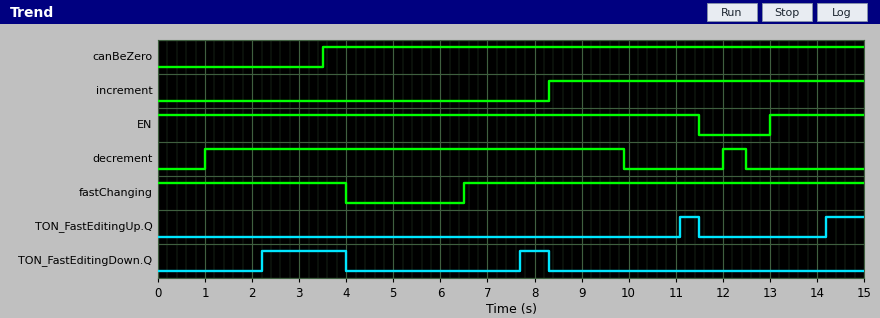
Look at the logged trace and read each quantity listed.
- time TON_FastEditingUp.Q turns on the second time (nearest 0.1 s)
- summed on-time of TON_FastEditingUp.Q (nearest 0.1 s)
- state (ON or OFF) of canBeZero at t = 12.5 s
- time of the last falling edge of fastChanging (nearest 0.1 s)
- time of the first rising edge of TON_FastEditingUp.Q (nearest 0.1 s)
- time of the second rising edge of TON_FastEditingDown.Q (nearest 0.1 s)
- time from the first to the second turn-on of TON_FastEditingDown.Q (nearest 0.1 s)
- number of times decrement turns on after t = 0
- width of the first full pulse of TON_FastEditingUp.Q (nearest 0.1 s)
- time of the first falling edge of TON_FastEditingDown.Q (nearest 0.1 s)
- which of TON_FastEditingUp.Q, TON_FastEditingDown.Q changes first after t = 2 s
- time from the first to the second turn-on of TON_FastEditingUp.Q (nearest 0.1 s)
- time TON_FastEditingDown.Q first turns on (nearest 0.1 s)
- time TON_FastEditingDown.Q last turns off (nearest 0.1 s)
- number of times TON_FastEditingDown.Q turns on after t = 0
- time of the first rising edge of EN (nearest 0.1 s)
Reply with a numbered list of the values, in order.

1. 14.2 s
2. 1.2 s
3. ON
4. 4.0 s
5. 11.1 s
6. 7.7 s
7. 5.5 s
8. 2
9. 0.4 s
10. 4.0 s
11. TON_FastEditingDown.Q
12. 3.1 s
13. 2.2 s
14. 8.3 s
15. 2
16. 13.0 s
